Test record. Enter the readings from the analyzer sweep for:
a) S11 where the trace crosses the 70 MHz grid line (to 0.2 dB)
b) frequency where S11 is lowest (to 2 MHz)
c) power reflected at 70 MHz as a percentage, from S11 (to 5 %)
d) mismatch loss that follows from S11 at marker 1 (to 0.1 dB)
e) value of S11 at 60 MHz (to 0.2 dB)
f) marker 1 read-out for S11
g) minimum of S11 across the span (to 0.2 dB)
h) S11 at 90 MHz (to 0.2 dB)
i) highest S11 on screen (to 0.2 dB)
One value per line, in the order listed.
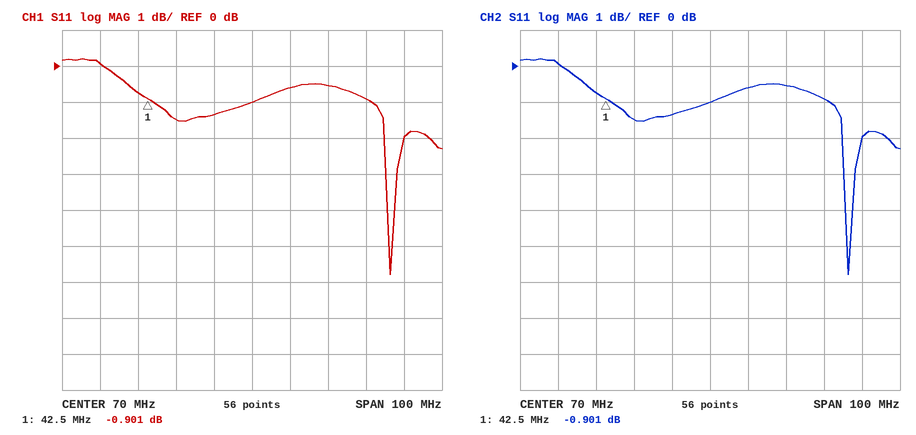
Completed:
-1.0 dB
106 MHz
80 %
7.3 dB
-1.4 dB
-0.901 dB
-5.8 dB
-0.6 dB
0.2 dB
